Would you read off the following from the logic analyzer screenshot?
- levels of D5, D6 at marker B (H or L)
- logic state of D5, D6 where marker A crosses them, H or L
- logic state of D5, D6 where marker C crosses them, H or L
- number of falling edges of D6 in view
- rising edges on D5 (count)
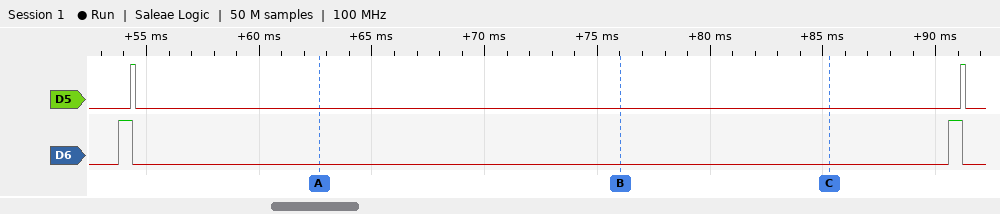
D5=L, D6=L
D5=L, D6=L
D5=L, D6=L
2
2
